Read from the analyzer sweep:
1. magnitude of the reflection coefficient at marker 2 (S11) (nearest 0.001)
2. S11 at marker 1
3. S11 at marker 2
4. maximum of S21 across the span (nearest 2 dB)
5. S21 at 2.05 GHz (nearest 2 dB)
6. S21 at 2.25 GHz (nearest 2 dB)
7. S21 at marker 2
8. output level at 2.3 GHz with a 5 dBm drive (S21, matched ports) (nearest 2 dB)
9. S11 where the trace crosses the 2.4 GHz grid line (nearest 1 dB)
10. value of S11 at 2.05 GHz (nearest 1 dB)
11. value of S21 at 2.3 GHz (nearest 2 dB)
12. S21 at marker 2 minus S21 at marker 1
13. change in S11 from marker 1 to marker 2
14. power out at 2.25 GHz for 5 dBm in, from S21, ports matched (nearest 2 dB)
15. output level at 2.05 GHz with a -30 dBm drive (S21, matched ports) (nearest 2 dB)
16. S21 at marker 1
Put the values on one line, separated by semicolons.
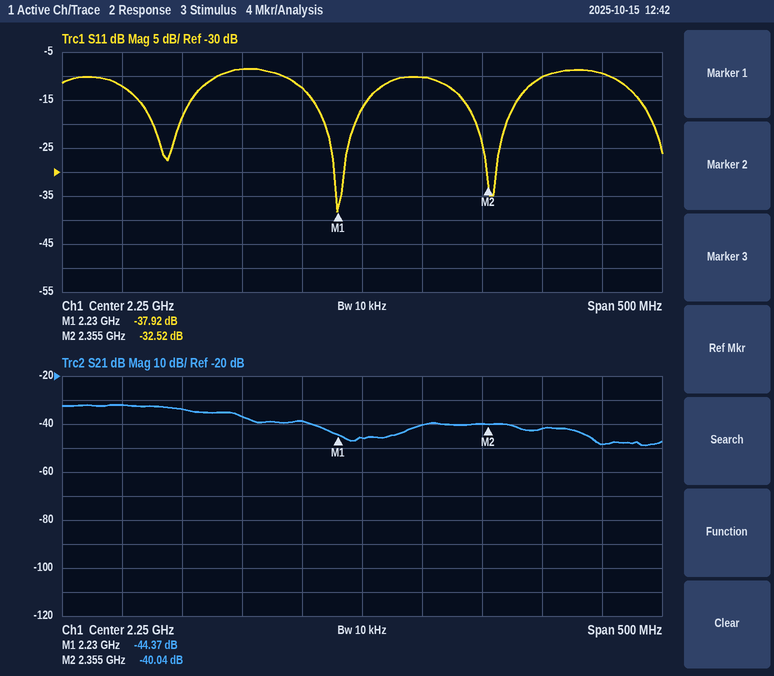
0.024; -37.92 dB; -32.52 dB; -32 dB; -32 dB; -46 dB; -40.04 dB; -36 dBm; -10 dB; -12 dB; -40 dB; 4.33 dB; 5.40 dB; -40 dBm; -62 dBm; -44.37 dB
